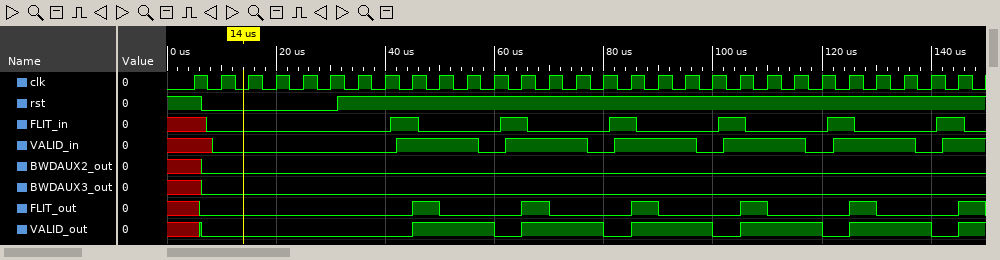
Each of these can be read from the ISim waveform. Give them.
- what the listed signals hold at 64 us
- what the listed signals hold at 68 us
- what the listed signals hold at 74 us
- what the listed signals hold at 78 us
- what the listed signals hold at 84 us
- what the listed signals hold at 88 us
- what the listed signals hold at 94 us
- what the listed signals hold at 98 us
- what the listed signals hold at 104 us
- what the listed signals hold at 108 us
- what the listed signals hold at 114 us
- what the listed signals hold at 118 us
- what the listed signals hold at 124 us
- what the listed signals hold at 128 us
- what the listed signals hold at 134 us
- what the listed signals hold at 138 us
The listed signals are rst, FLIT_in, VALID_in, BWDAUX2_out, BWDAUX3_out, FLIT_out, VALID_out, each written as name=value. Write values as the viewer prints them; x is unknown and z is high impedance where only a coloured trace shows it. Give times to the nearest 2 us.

rst=1, FLIT_in=1, VALID_in=1, BWDAUX2_out=0, BWDAUX3_out=0, FLIT_out=0, VALID_out=0
rst=1, FLIT_in=0, VALID_in=1, BWDAUX2_out=0, BWDAUX3_out=0, FLIT_out=1, VALID_out=1
rst=1, FLIT_in=0, VALID_in=1, BWDAUX2_out=0, BWDAUX3_out=0, FLIT_out=0, VALID_out=1
rst=1, FLIT_in=0, VALID_in=0, BWDAUX2_out=0, BWDAUX3_out=0, FLIT_out=0, VALID_out=1
rst=1, FLIT_in=1, VALID_in=1, BWDAUX2_out=0, BWDAUX3_out=0, FLIT_out=0, VALID_out=0
rst=1, FLIT_in=0, VALID_in=1, BWDAUX2_out=0, BWDAUX3_out=0, FLIT_out=1, VALID_out=1
rst=1, FLIT_in=0, VALID_in=1, BWDAUX2_out=0, BWDAUX3_out=0, FLIT_out=0, VALID_out=1
rst=1, FLIT_in=0, VALID_in=0, BWDAUX2_out=0, BWDAUX3_out=0, FLIT_out=0, VALID_out=1
rst=1, FLIT_in=1, VALID_in=1, BWDAUX2_out=0, BWDAUX3_out=0, FLIT_out=0, VALID_out=0
rst=1, FLIT_in=0, VALID_in=1, BWDAUX2_out=0, BWDAUX3_out=0, FLIT_out=1, VALID_out=1
rst=1, FLIT_in=0, VALID_in=1, BWDAUX2_out=0, BWDAUX3_out=0, FLIT_out=0, VALID_out=1
rst=1, FLIT_in=0, VALID_in=0, BWDAUX2_out=0, BWDAUX3_out=0, FLIT_out=0, VALID_out=1
rst=1, FLIT_in=1, VALID_in=1, BWDAUX2_out=0, BWDAUX3_out=0, FLIT_out=0, VALID_out=0
rst=1, FLIT_in=0, VALID_in=1, BWDAUX2_out=0, BWDAUX3_out=0, FLIT_out=1, VALID_out=1
rst=1, FLIT_in=0, VALID_in=1, BWDAUX2_out=0, BWDAUX3_out=0, FLIT_out=0, VALID_out=1
rst=1, FLIT_in=0, VALID_in=0, BWDAUX2_out=0, BWDAUX3_out=0, FLIT_out=0, VALID_out=1
